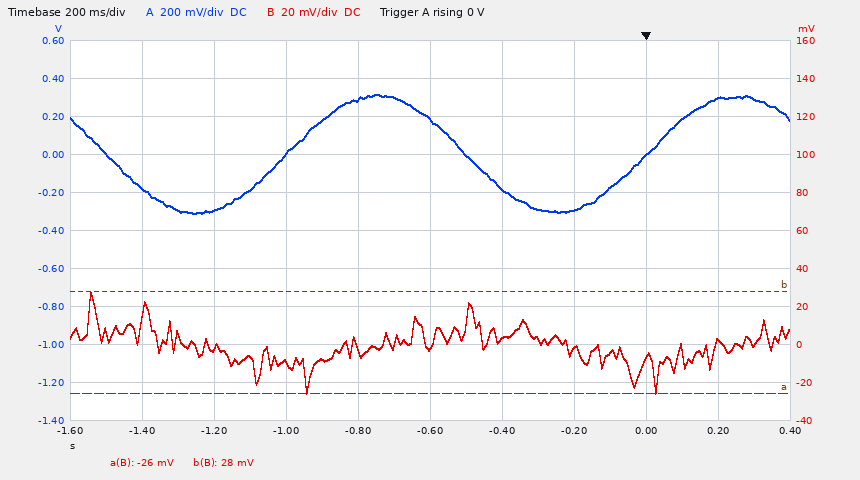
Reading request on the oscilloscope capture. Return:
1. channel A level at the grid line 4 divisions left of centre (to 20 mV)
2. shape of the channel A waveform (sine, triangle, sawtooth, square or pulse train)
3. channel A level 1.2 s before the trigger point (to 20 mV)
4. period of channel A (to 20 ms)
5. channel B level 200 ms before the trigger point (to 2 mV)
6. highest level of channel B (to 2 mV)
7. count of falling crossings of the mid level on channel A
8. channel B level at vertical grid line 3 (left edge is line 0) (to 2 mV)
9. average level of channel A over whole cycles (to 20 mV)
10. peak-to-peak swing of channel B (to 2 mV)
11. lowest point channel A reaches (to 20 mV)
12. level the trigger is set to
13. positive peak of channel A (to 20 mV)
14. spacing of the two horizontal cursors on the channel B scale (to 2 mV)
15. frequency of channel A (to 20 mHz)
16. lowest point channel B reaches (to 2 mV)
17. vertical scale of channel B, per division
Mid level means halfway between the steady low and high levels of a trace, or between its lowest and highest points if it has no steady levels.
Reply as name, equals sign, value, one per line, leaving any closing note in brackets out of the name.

channel A level at the grid line 4 divisions left of centre = -180 mV
shape of the channel A waveform = sine
channel A level 1.2 s before the trigger point = -300 mV
period of channel A = 1.00 s
channel B level 200 ms before the trigger point = -2 mV
highest level of channel B = 28 mV
count of falling crossings of the mid level on channel A = 2
channel B level at vertical grid line 3 (left edge is line 0) = -10 mV
average level of channel A over whole cycles = 0 mV
peak-to-peak swing of channel B = 54 mV
lowest point channel A reaches = -320 mV
level the trigger is set to = 0 V
positive peak of channel A = 320 mV
spacing of the two horizontal cursors on the channel B scale = 54 mV
frequency of channel A = 1.00 Hz
lowest point channel B reaches = -26 mV
vertical scale of channel B, per division = 20 mV
